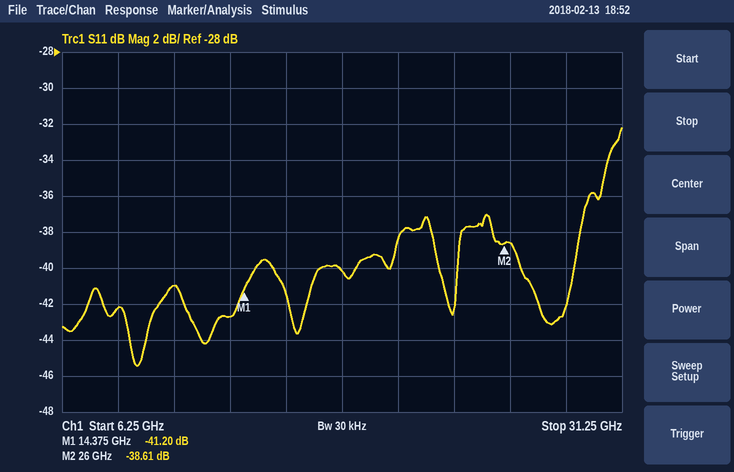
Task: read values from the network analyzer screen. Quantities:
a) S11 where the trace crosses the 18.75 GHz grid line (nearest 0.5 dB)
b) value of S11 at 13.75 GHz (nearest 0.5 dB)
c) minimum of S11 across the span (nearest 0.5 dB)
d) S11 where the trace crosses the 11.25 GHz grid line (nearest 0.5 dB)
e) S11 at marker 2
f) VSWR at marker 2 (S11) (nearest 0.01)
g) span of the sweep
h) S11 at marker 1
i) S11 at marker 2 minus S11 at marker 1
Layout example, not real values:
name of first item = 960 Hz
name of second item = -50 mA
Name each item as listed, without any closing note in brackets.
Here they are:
S11 where the trace crosses the 18.75 GHz grid line = -40.0 dB
value of S11 at 13.75 GHz = -42.5 dB
minimum of S11 across the span = -45.5 dB
S11 where the trace crosses the 11.25 GHz grid line = -41.0 dB
S11 at marker 2 = -38.61 dB
VSWR at marker 2 (S11) = 1.02
span of the sweep = 25 GHz
S11 at marker 1 = -41.20 dB
S11 at marker 2 minus S11 at marker 1 = 2.59 dB
